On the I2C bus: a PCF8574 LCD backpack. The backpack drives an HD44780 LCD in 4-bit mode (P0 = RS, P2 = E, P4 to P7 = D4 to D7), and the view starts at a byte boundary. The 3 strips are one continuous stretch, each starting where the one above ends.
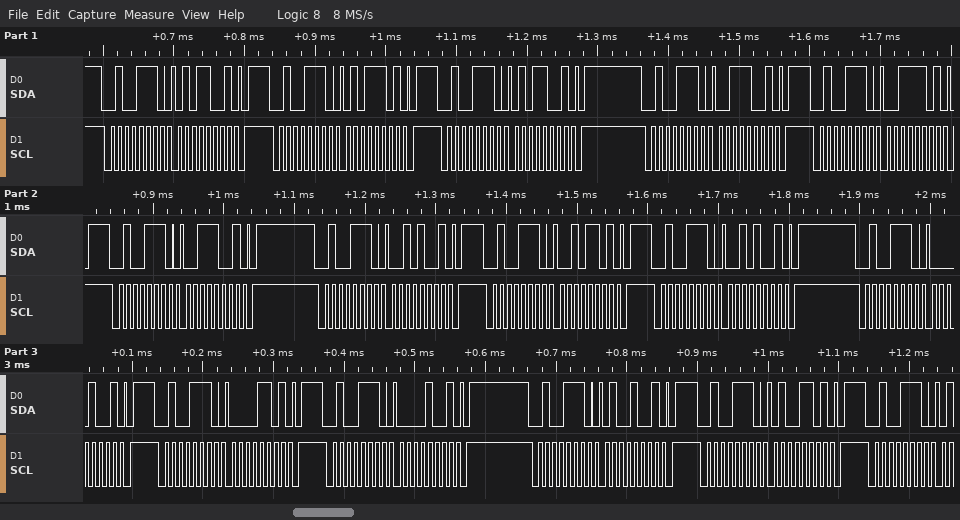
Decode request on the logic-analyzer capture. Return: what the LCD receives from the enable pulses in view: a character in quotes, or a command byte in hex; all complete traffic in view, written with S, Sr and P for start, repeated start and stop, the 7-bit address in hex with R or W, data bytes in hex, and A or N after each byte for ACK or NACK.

'S' ' '
S 27W A 59 A P S 27W A 5D A P S 27W A 59 A P S 27W A 39 A P S 27W A 3D A P S 27W A 39 A P S 27W A 29 A P S 27W A 2D A P S 27W A 29 A P S 27W A 09 A P S 27W A 0D A P S 27W A 09 A P S 27W A 49 A P S 27W A 4D A P S 27W A
